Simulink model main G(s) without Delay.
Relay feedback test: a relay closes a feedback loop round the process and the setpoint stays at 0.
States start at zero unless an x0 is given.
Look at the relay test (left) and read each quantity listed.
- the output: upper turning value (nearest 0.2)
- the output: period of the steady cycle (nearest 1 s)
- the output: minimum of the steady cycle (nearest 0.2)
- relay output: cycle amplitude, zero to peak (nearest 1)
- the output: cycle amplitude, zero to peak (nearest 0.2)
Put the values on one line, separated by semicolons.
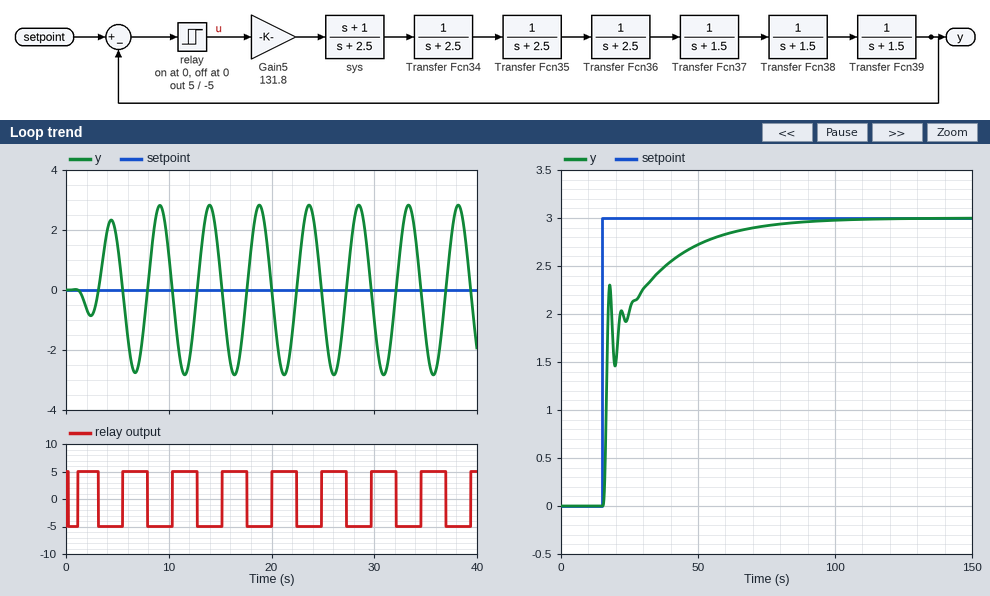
2.8; 5 s; -2.8; 5; 2.8
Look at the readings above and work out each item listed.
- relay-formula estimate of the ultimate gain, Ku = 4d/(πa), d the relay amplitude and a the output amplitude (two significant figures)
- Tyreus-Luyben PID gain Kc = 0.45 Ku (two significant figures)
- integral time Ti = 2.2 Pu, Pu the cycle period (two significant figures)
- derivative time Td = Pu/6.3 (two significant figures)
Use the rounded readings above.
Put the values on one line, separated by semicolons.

2.3; 1.0; 11 s; 0.79 s
